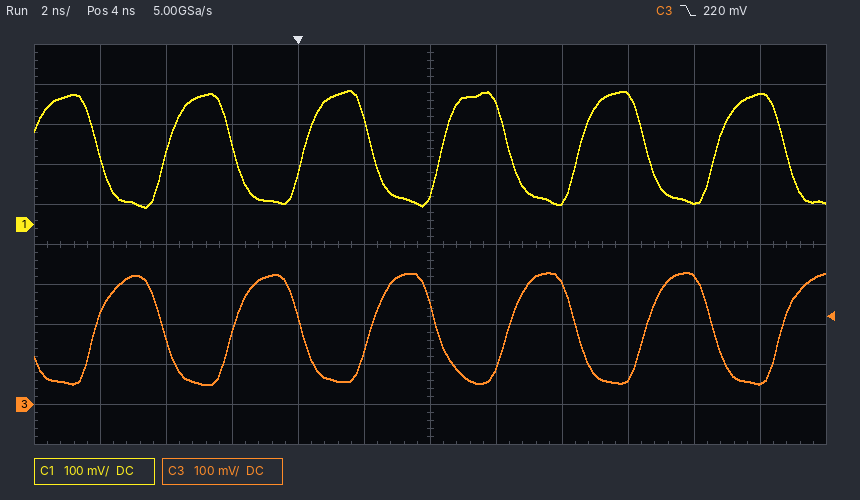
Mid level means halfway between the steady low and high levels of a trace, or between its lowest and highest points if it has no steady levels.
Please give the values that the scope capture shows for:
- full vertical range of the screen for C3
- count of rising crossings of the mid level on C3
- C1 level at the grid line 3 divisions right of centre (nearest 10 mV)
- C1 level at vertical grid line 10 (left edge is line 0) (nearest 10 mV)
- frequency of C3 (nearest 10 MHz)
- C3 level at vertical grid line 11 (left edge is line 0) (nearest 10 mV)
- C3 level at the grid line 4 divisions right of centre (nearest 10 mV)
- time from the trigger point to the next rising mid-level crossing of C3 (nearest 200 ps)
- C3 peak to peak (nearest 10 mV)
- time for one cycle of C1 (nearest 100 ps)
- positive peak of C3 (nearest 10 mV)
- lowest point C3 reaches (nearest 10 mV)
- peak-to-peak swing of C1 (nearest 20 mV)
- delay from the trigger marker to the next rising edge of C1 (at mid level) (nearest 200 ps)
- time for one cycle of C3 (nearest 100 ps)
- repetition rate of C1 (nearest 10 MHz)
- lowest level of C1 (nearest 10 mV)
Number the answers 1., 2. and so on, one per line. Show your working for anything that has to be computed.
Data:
1. 1 V
2. 6
3. 320 mV
4. 50 mV
5. 1 / 4.2 ns ≈ 238 MHz, so 240 MHz to the nearest 10 MHz
6. 50 mV
7. 320 mV
8. 2.2 ns
9. 330 mV − (50 mV) = 280 mV
10. 4.2 ns
11. 330 mV
12. 50 mV
13. 300 mV
14. 200 ps
15. 4.2 ns
16. 1 / 4.2 ns ≈ 238 MHz, so 240 MHz to the nearest 10 MHz
17. 40 mV
